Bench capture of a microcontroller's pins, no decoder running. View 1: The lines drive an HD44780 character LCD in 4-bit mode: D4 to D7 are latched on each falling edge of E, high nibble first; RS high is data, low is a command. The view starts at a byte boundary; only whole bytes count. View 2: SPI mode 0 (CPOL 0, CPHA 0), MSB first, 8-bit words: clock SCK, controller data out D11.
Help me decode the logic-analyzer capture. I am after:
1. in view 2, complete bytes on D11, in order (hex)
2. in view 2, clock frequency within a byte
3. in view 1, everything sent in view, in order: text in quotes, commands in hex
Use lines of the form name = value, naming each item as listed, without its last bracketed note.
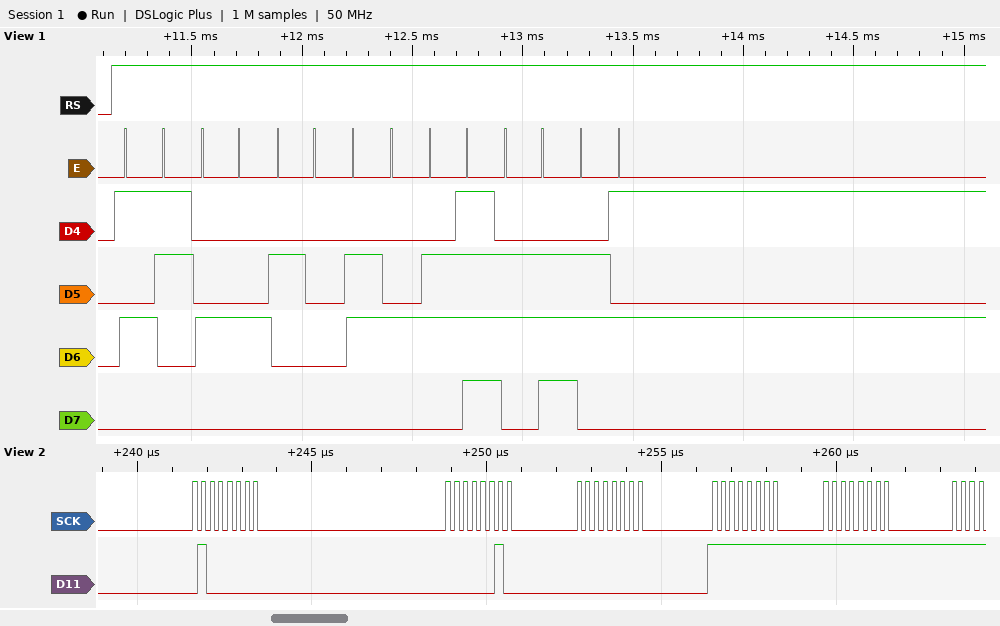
in view 2, complete bytes on D11, in order = 40 02 00 FF FF
in view 2, clock frequency within a byte = 4 MHz
in view 1, everything sent in view, in order: text in quotes, commands in hex = "SD done"
